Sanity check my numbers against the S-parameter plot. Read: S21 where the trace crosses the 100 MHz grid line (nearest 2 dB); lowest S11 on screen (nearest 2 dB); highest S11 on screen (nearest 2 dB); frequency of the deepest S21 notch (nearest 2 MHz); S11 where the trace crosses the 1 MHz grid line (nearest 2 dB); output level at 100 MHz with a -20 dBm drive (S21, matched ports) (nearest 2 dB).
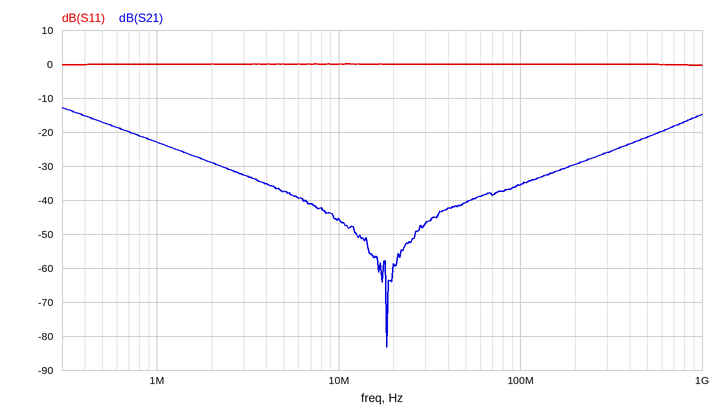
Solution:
-36 dB
0 dB
0 dB
18 MHz
0 dB
-56 dBm
